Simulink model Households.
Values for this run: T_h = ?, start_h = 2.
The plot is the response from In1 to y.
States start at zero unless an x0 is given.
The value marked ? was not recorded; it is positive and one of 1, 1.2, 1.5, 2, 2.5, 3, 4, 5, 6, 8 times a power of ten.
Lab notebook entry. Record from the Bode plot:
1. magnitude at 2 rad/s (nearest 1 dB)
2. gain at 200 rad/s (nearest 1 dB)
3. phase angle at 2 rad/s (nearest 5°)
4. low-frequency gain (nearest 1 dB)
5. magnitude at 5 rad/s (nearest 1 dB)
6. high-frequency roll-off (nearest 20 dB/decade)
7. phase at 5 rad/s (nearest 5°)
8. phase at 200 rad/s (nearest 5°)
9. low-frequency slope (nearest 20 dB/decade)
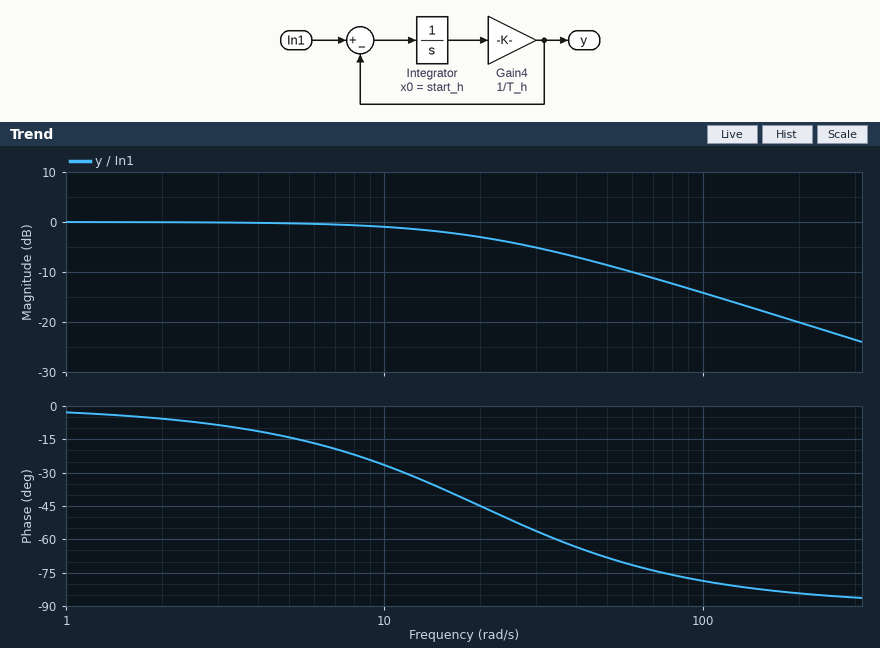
0 dB
-20 dB
-5°
0 dB
0 dB
-20 dB/decade
-15°
-85°
0 dB/decade
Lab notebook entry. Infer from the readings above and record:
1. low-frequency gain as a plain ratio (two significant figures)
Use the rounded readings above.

1.0
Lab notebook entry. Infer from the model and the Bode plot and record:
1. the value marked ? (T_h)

0.05
